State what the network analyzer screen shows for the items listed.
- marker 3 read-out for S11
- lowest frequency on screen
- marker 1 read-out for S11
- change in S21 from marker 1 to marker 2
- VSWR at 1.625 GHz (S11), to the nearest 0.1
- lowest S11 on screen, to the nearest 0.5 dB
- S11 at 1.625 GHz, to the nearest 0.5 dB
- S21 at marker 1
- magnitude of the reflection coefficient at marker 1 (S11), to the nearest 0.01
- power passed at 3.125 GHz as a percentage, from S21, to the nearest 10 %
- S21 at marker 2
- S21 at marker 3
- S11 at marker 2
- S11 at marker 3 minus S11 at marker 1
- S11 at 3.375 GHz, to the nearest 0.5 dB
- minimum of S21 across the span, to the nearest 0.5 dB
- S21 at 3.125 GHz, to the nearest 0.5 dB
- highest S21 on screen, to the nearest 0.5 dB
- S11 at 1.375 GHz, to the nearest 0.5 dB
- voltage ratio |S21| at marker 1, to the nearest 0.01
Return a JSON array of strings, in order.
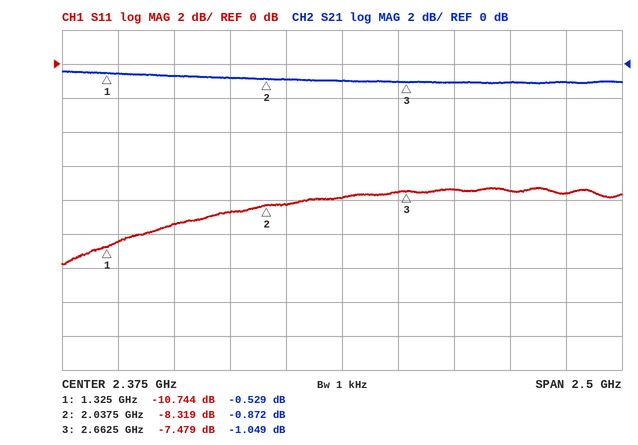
["-7.479 dB", "1.125 GHz", "-10.744 dB", "-0.343 dB", "2.0", "-12.0 dB", "-9.5 dB", "-0.529 dB", "0.29", "80 %", "-0.872 dB", "-1.049 dB", "-8.319 dB", "3.265 dB", "-7.5 dB", "-1.0 dB", "-1.0 dB", "-0.5 dB", "-10.5 dB", "0.94"]
